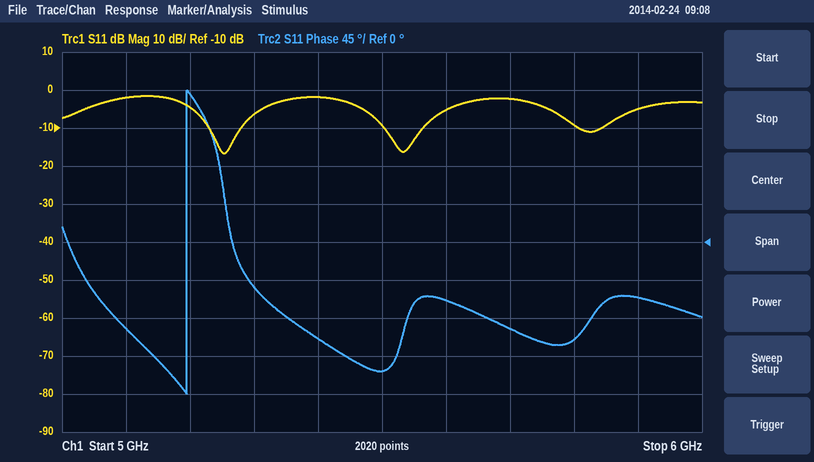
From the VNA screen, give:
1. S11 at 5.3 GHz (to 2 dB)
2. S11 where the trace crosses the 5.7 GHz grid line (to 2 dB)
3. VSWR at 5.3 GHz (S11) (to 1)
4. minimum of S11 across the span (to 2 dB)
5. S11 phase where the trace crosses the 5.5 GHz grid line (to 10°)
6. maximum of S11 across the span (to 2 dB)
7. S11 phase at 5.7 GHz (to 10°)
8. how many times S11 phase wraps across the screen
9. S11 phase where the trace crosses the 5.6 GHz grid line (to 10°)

-6 dB
-2 dB
3
-16 dB
-150°
-2 dB
-100°
1
-70°
